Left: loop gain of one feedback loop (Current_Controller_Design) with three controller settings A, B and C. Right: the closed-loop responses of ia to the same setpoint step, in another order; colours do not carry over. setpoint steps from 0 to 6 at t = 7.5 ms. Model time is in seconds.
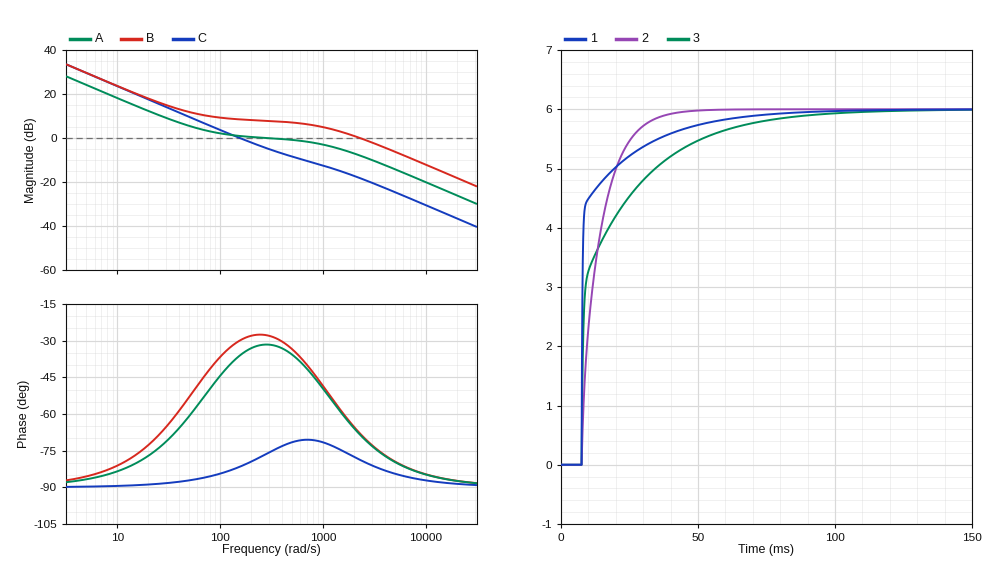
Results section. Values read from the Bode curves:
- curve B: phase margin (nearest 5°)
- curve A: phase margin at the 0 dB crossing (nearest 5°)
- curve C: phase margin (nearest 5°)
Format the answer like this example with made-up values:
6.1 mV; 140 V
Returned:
110°; 150°; 100°
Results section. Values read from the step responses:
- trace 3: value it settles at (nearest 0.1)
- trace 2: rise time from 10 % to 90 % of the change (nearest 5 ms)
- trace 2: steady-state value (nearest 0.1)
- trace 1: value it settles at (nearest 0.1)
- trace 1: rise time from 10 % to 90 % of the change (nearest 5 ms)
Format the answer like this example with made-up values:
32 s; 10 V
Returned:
6.0; 15 ms; 6.0; 6.0; 25 ms
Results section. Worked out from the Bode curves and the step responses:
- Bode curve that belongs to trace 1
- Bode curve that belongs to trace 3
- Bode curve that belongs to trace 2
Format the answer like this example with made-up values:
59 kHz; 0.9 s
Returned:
B; A; C
